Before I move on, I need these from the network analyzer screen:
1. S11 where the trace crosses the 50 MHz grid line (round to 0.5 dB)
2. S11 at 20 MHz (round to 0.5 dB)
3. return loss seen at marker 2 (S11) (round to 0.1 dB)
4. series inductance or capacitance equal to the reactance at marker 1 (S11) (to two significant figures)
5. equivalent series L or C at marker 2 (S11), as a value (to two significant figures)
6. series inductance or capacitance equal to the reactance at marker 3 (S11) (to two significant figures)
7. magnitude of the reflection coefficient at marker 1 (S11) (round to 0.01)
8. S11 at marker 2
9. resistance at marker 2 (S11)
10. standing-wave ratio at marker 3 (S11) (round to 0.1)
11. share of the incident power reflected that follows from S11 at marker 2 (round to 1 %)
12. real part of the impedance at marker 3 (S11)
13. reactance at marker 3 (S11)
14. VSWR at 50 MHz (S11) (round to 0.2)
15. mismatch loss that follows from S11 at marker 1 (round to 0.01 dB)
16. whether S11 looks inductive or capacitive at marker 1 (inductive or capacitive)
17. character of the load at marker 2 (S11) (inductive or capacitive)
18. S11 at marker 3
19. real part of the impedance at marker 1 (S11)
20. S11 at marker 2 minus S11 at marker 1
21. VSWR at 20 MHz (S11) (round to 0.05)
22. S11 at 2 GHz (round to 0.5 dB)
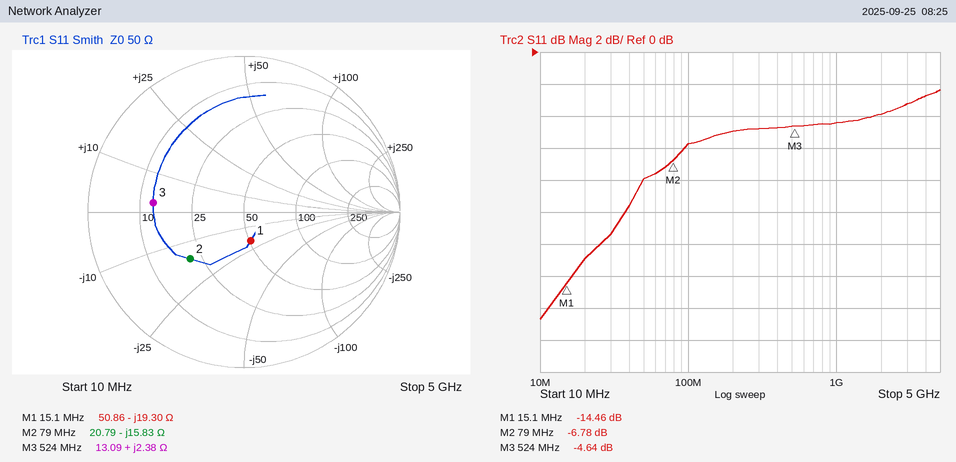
-8.0 dB
-13.0 dB
6.8 dB
550 pF
130 pF
720 pH
0.19
-6.78 dB
20.79 Ω
3.8
21 %
13.09 Ω
+2.38 Ω
2.4
0.16 dB
capacitive
capacitive
-4.64 dB
50.86 Ω
7.68 dB
1.60
-4.0 dB
